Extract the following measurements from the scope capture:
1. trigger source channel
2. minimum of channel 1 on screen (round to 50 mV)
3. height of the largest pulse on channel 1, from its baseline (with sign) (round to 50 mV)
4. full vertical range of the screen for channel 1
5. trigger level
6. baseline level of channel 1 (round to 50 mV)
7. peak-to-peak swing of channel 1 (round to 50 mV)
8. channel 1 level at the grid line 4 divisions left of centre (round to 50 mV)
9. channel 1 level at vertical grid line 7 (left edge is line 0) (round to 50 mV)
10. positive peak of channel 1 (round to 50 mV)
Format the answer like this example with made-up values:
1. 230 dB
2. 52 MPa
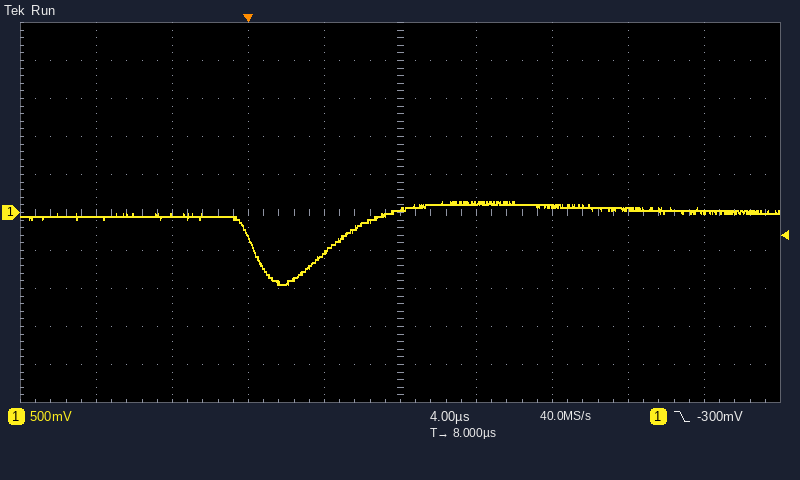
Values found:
1. channel 1
2. -950 mV
3. -900 mV
4. 5 V
5. -300 mV
6. -50 mV
7. 1.10 V
8. -50 mV
9. 100 mV
10. 150 mV
